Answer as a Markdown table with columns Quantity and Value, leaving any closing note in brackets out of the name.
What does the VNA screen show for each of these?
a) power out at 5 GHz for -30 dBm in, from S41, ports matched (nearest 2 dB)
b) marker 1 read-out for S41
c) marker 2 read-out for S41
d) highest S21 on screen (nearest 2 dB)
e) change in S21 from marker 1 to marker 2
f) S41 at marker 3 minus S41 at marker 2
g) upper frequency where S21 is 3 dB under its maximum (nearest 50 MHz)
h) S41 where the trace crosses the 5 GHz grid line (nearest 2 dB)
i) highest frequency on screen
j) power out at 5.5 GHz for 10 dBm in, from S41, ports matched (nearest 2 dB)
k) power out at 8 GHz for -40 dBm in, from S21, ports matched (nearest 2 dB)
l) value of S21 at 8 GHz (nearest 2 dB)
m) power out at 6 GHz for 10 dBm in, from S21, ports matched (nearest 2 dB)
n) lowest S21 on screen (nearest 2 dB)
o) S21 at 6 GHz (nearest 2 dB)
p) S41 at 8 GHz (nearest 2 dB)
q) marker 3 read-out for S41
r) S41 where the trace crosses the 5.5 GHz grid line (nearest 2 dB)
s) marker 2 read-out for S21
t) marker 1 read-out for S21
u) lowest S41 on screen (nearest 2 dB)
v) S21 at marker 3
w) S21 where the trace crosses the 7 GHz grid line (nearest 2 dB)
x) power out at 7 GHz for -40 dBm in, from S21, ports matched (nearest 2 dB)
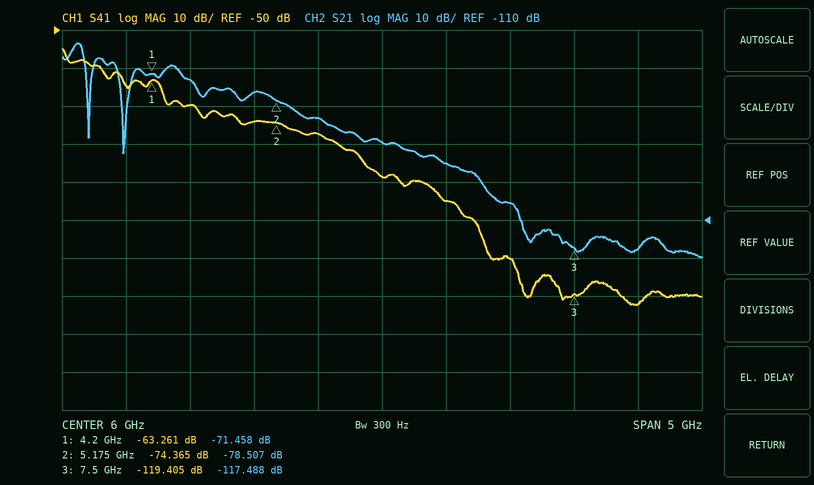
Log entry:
| Quantity | Value |
|---|---|
| power out at 5 GHz for -30 dBm in, from S41, ports matched | -104 dBm |
| marker 1 read-out for S41 | -63.261 dB |
| marker 2 read-out for S41 | -74.365 dB |
| highest S21 on screen | -64 dB |
| change in S21 from marker 1 to marker 2 | -7.049 dB |
| S41 at marker 3 minus S41 at marker 2 | -45.040 dB |
| upper frequency where S21 is 3 dB under its maximum | 3.65 GHz |
| S41 where the trace crosses the 5 GHz grid line | -74 dB |
| highest frequency on screen | 8.5 GHz |
| power out at 5.5 GHz for 10 dBm in, from S41, ports matched | -68 dBm |
| power out at 8 GHz for -40 dBm in, from S21, ports matched | -158 dBm |
| value of S21 at 8 GHz | -118 dB |
| power out at 6 GHz for 10 dBm in, from S21, ports matched | -80 dBm |
| lowest S21 on screen | -120 dB |
| S21 at 6 GHz | -90 dB |
| S41 at 8 GHz | -122 dB |
| marker 3 read-out for S41 | -119.405 dB |
| S41 where the trace crosses the 5.5 GHz grid line | -78 dB |
| marker 2 read-out for S21 | -78.507 dB |
| marker 1 read-out for S21 | -71.458 dB |
| lowest S41 on screen | -122 dB |
| S21 at marker 3 | -117.488 dB |
| S21 where the trace crosses the 7 GHz grid line | -106 dB |
| power out at 7 GHz for -40 dBm in, from S21, ports matched | -146 dBm |
